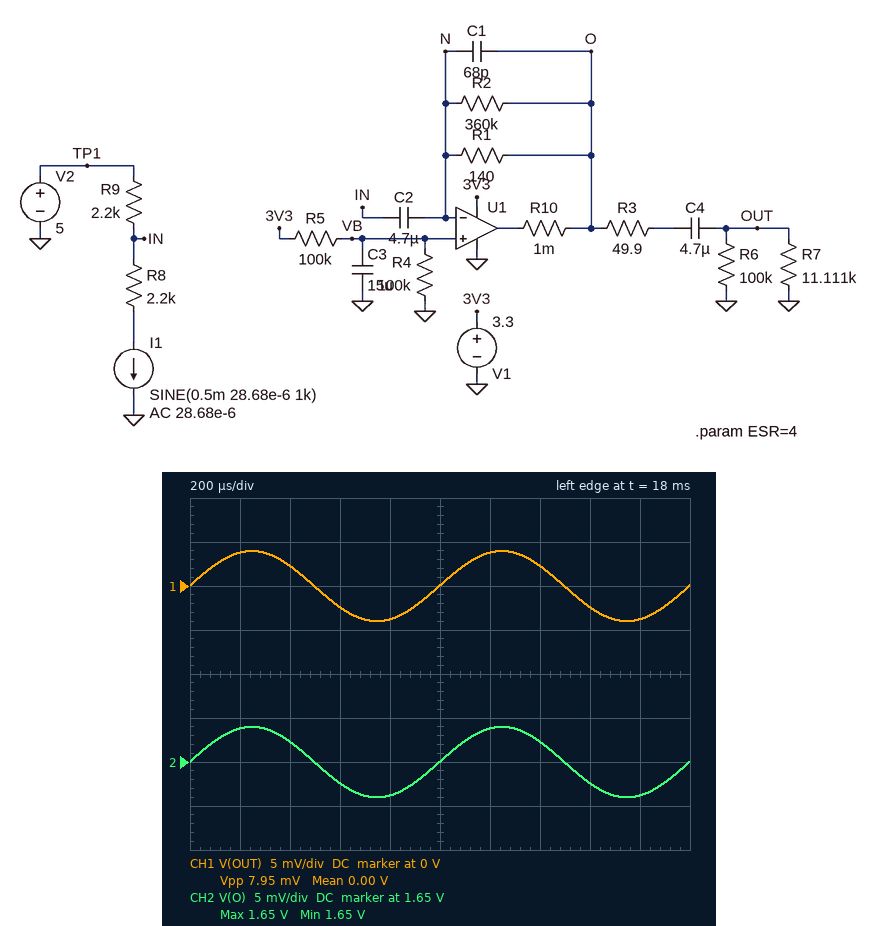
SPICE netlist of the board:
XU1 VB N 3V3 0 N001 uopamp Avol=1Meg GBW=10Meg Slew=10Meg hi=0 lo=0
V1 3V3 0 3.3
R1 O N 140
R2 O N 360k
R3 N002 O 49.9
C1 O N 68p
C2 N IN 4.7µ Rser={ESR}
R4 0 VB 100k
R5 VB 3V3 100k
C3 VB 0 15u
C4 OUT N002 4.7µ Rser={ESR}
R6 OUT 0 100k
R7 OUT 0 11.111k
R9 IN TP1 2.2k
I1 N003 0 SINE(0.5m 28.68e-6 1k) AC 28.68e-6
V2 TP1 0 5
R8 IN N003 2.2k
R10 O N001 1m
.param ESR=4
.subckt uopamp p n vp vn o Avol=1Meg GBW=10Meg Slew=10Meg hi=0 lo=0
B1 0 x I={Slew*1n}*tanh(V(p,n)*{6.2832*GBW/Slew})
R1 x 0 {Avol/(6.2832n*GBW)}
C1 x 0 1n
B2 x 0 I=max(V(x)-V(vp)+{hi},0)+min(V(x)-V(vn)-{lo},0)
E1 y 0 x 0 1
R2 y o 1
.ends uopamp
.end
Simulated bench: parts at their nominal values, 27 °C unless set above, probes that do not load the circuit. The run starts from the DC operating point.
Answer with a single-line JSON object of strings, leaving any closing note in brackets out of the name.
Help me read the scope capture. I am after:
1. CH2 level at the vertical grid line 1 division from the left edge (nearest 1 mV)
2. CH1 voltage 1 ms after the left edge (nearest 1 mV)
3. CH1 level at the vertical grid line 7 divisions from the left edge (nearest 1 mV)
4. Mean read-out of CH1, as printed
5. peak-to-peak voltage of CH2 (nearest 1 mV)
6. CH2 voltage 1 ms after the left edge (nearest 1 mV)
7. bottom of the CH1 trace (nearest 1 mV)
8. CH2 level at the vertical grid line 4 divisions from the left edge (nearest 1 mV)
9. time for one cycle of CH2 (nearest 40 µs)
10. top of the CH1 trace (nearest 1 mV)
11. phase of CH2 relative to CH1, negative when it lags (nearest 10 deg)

{"CH2 level at the vertical grid line 1 division from the left edge": "1.654 V", "CH1 voltage 1 ms after the left edge": "0 V", "CH1 level at the vertical grid line 7 divisions from the left edge": "2 mV", "Mean read-out of CH1, as printed": "0.00 V", "peak-to-peak voltage of CH2": "8 mV", "CH2 voltage 1 ms after the left edge": "1.650 V", "bottom of the CH1 trace": "-4 mV", "CH2 level at the vertical grid line 4 divisions from the left edge": "1.646 V", "time for one cycle of CH2": "1.00 ms", "top of the CH1 trace": "4 mV", "phase of CH2 relative to CH1, negative when it lags": "0 deg"}
